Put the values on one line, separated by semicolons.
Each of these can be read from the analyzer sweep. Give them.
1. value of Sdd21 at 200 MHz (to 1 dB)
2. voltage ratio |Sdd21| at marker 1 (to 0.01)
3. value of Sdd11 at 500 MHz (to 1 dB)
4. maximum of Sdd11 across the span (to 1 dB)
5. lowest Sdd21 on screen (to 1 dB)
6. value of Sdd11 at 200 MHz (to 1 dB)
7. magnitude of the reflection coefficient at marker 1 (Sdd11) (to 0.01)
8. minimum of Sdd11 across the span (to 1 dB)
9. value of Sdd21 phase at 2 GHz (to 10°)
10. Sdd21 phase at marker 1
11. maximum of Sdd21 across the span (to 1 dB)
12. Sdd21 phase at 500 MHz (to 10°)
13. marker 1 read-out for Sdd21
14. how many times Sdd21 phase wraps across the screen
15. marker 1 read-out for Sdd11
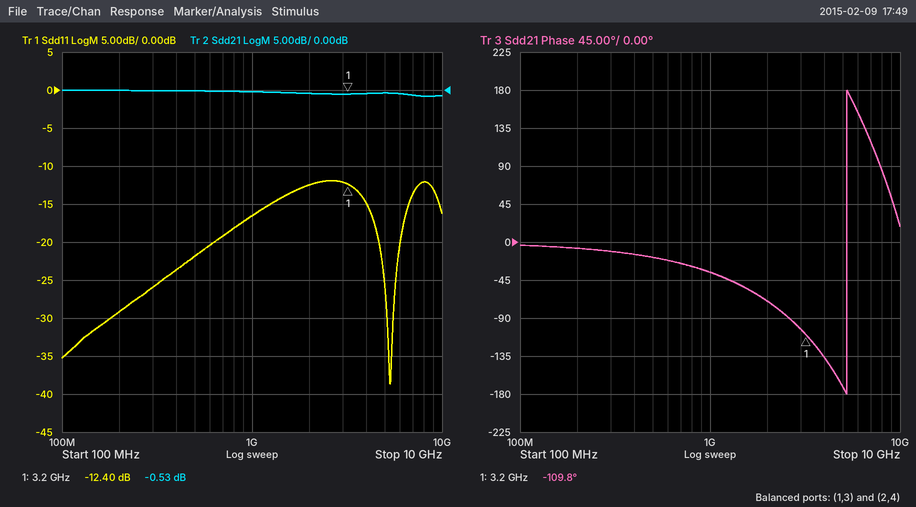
0 dB; 0.94; -22 dB; -12 dB; -1 dB; -29 dB; 0.24; -39 dB; -70°; -109.8°; 0 dB; -20°; -0.53 dB; 1; -12.40 dB
